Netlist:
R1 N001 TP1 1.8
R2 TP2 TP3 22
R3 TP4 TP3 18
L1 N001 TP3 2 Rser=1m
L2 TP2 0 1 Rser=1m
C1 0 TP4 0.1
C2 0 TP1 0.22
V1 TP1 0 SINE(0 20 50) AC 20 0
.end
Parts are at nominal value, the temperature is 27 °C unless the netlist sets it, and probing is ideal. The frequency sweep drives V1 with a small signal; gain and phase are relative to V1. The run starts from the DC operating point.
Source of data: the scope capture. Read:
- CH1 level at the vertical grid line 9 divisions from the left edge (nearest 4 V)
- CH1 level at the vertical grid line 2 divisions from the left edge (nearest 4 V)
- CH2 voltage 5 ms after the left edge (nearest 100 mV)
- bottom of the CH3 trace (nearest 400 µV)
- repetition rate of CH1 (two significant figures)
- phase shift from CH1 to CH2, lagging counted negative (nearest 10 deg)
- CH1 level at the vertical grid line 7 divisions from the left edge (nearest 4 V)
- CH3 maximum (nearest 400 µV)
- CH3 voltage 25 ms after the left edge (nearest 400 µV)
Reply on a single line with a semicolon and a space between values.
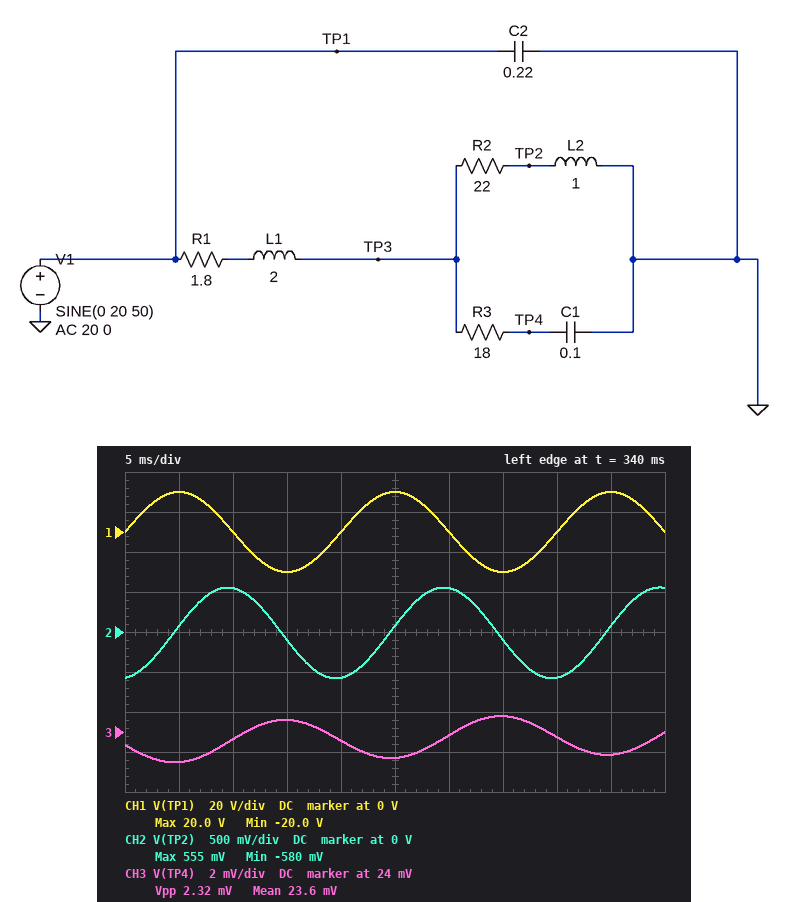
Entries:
20 V; 0 V; 100 mV; 22.4 mV; 50 Hz; -80 deg; -20 V; 24.8 mV; 22.8 mV
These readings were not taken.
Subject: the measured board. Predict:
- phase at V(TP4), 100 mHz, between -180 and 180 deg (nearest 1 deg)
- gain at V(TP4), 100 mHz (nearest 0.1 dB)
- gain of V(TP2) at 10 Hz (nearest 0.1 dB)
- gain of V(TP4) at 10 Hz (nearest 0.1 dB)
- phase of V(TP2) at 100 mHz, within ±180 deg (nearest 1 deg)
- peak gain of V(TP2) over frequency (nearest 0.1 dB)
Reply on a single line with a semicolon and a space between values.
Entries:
-56 deg; -4.5 dB; -18.7 dB; -59.2 dB; 81 deg; -14.8 dB
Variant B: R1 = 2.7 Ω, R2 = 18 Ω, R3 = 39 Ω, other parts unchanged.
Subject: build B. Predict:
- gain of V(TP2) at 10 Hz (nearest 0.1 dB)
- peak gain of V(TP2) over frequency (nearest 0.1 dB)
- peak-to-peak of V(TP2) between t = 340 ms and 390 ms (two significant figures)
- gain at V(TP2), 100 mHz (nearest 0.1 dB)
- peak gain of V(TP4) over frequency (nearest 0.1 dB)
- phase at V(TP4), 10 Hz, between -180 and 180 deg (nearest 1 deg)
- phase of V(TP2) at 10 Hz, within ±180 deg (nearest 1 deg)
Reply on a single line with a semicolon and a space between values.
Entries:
-13.8 dB; -12.0 dB; 2.4 V; -30.8 dB; -1.2 dB; -142 deg; -36 deg
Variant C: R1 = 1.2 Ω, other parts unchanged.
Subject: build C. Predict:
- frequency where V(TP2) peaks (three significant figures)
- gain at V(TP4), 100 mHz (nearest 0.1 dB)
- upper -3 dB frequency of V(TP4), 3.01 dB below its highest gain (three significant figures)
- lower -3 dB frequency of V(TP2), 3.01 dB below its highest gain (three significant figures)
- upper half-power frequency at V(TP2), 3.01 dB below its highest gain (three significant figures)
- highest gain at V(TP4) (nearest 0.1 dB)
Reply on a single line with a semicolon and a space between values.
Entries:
2.31 Hz; -4.1 dB; 86.8 mHz; 630 mHz; 8.44 Hz; -0.5 dB
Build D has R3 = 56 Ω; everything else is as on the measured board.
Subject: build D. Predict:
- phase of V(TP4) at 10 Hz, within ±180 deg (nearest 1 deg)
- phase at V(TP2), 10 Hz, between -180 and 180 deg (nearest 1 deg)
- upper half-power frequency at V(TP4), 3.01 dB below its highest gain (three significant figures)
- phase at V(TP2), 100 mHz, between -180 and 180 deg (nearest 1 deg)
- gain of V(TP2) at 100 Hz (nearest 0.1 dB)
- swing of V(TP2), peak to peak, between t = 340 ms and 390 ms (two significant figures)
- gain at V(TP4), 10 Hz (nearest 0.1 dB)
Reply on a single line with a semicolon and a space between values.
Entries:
-135 deg; -26 deg; 27.7 mHz; 84 deg; -27.1 dB; 3.4 V; -63.0 dB
